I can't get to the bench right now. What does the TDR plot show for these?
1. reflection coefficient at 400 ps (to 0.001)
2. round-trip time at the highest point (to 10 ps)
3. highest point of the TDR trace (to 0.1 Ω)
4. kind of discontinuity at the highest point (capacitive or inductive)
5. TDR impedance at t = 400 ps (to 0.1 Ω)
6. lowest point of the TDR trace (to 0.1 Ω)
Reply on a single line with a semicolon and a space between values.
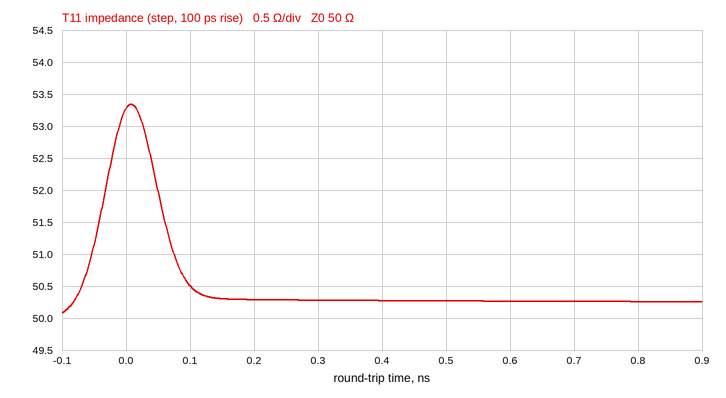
+0.003; 10 ps; 53.3 Ω; inductive; 50.3 Ω; 50.1 Ω
